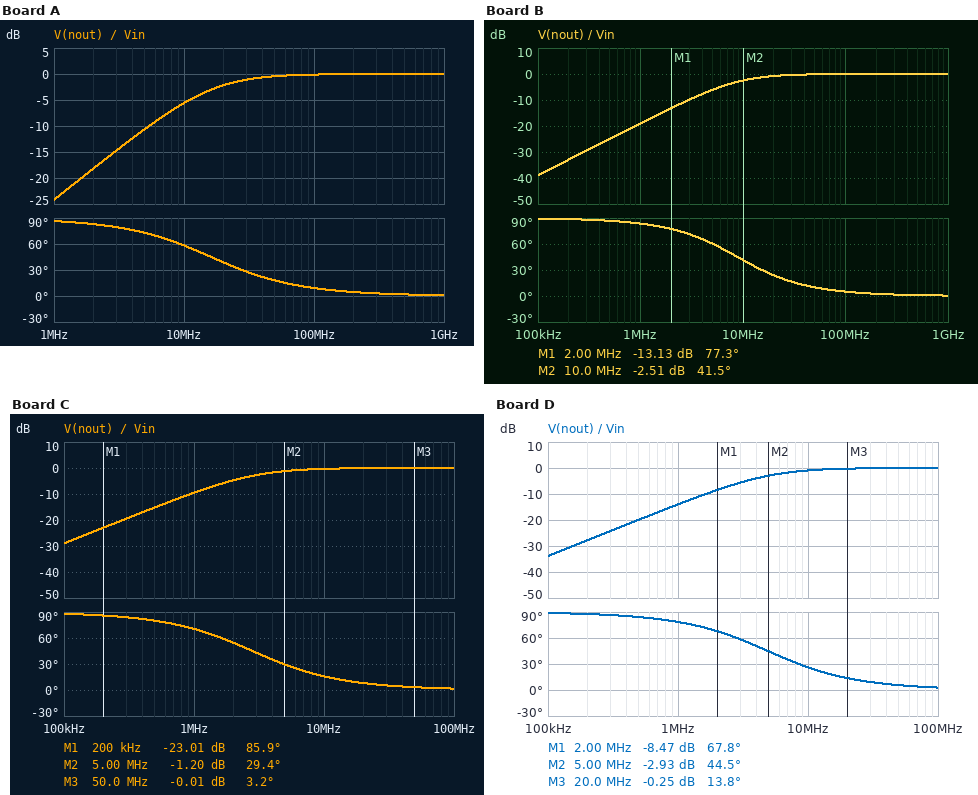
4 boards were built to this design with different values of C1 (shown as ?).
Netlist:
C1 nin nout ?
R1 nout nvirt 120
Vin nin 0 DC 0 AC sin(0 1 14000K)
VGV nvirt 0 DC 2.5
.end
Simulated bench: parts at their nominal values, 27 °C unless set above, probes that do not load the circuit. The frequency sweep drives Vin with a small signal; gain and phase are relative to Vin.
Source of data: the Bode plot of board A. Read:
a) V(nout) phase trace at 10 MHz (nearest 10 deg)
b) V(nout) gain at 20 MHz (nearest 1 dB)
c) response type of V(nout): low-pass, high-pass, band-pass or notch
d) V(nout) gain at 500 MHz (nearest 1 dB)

60 deg
-2 dB
high-pass
0 dB
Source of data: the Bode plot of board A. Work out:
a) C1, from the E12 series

82 pF
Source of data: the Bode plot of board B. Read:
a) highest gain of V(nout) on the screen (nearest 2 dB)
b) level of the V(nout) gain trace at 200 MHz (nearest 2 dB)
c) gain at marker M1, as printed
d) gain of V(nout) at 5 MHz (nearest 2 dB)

0 dB
0 dB
-13.13 dB
-6 dB
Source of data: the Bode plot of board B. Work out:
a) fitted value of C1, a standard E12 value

150 pF
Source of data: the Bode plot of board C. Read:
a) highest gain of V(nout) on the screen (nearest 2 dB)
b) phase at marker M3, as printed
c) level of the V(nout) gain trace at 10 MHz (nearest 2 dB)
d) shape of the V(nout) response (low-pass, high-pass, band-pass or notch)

0 dB
3.2 deg
0 dB
high-pass
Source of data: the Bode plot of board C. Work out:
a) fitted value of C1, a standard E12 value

470 pF
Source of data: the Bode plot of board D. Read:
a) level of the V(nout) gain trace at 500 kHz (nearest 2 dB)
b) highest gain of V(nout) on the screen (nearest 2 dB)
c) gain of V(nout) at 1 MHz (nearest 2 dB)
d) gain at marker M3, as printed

-20 dB
0 dB
-14 dB
-0.25 dB
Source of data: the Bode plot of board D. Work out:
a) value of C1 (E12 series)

270 pF
